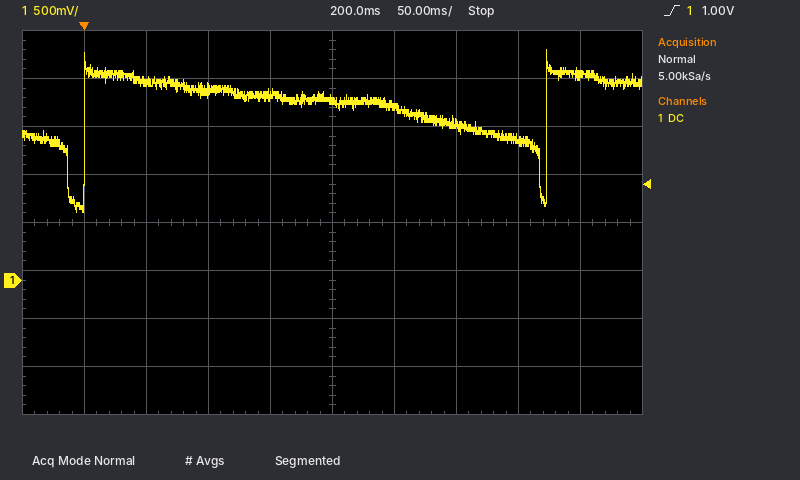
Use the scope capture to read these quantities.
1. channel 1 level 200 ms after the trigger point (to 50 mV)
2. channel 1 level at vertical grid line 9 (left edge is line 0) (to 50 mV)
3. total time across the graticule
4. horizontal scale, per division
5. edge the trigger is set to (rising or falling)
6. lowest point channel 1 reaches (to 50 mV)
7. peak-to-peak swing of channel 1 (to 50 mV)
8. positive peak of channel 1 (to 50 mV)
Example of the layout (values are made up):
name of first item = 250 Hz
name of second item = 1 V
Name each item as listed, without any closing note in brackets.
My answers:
channel 1 level 200 ms after the trigger point = 1.90 V
channel 1 level at vertical grid line 9 (left edge is line 0) = 2.15 V
total time across the graticule = 500 ms
horizontal scale, per division = 50 ms
edge the trigger is set to = rising
lowest point channel 1 reaches = 700 mV
peak-to-peak swing of channel 1 = 1.70 V
positive peak of channel 1 = 2.40 V
